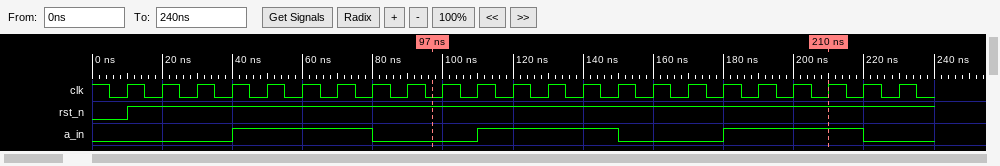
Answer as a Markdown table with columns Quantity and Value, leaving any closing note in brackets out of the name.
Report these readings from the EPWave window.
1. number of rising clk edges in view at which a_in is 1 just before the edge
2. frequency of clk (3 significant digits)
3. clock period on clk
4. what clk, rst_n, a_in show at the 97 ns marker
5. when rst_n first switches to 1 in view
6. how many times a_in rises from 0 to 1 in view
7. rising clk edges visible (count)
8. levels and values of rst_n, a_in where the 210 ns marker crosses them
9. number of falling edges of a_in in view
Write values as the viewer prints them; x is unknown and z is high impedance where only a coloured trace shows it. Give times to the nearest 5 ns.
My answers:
| Quantity | Value |
|---|---|
| number of rising clk edges in view at which a_in is 1 just before the edge | 12 |
| frequency of clk | 100 MHz |
| clock period on clk | 10 ns |
| what clk, rst_n, a_in show at the 97 ns marker | clk=0, rst_n=1, a_in=0 |
| when rst_n first switches to 1 in view | 10 ns |
| how many times a_in rises from 0 to 1 in view | 3 |
| rising clk edges visible | 23 |
| levels and values of rst_n, a_in where the 210 ns marker crosses them | rst_n=1, a_in=1 |
| number of falling edges of a_in in view | 3 |
